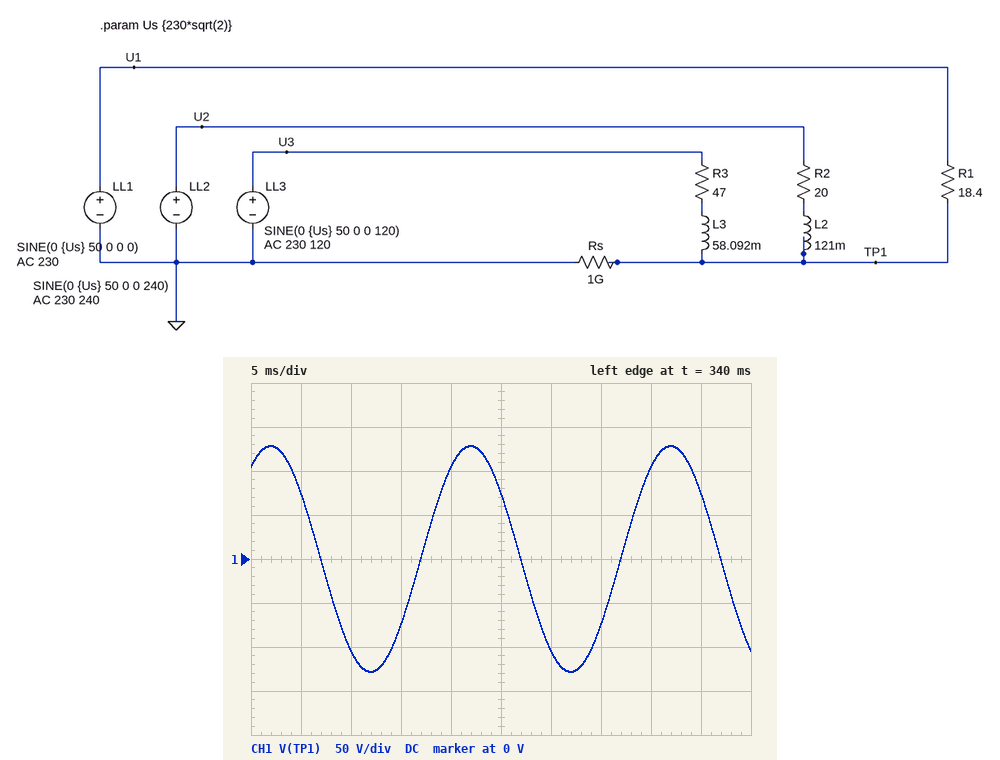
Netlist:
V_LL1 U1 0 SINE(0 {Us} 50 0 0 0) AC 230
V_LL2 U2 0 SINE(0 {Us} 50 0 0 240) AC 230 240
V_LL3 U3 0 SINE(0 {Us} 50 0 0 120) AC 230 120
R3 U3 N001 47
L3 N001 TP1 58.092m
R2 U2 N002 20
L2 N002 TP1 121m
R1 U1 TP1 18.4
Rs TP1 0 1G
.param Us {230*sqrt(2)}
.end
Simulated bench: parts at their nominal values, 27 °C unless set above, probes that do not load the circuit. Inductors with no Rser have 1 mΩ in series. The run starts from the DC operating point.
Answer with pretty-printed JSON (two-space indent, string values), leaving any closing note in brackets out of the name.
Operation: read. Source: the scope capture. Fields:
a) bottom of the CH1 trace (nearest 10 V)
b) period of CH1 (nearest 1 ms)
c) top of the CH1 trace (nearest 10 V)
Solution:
{
  "bottom of the CH1 trace": "-130 V",
  "period of CH1": "20 ms",
  "top of the CH1 trace": "130 V"
}
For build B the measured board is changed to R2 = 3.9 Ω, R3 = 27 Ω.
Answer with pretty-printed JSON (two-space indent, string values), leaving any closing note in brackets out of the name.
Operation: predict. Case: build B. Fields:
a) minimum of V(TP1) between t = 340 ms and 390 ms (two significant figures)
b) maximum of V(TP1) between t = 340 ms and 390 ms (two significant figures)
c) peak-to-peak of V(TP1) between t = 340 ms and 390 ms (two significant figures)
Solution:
{
  "minimum of V(TP1) between t = 340 ms and 390 ms": "-180 V",
  "maximum of V(TP1) between t = 340 ms and 390 ms": "180 V",
  "peak-to-peak of V(TP1) between t = 340 ms and 390 ms": "370 V"
}
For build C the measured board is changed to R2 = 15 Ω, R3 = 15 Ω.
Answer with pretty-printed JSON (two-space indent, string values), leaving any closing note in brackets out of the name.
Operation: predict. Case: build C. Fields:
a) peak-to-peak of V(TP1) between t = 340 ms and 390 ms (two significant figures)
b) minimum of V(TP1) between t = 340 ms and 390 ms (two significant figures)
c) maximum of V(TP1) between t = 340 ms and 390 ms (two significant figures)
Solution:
{
  "peak-to-peak of V(TP1) between t = 340 ms and 390 ms": "380 V",
  "minimum of V(TP1) between t = 340 ms and 390 ms": "-190 V",
  "maximum of V(TP1) between t = 340 ms and 390 ms": "190 V"
}
